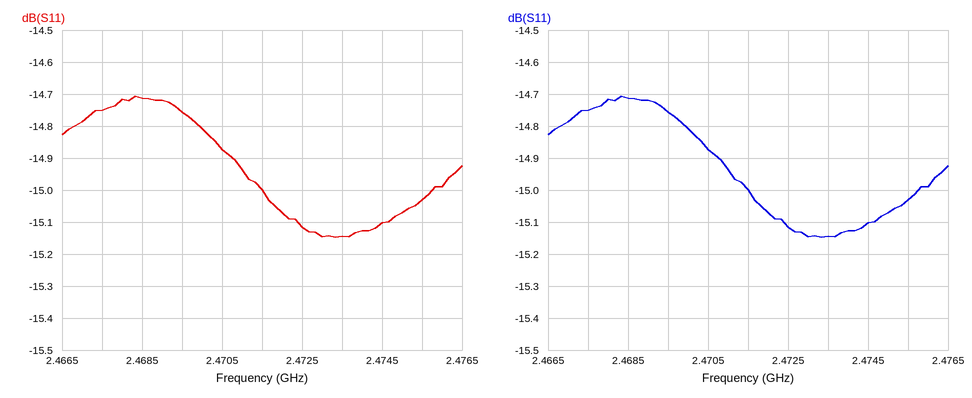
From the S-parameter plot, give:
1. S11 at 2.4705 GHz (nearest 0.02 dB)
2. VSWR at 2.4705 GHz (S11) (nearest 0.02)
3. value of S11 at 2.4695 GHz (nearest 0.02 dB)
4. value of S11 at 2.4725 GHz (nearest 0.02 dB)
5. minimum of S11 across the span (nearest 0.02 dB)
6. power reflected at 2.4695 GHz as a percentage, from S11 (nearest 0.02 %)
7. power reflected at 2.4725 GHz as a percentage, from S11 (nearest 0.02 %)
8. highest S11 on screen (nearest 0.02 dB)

-14.88 dB
1.44
-14.76 dB
-15.12 dB
-15.14 dB
3.34 %
3.08 %
-14.70 dB
